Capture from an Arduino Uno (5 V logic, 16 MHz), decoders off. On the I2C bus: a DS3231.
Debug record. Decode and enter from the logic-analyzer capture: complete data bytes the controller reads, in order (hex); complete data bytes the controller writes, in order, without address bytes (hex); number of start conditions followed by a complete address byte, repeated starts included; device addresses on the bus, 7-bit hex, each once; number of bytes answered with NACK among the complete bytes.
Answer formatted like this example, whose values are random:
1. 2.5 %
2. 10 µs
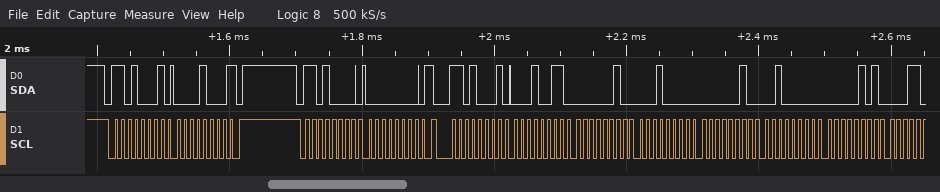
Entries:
1. 08 13 02 10 02 20 05
2. 00
3. 3
4. 0x68
5. 1
